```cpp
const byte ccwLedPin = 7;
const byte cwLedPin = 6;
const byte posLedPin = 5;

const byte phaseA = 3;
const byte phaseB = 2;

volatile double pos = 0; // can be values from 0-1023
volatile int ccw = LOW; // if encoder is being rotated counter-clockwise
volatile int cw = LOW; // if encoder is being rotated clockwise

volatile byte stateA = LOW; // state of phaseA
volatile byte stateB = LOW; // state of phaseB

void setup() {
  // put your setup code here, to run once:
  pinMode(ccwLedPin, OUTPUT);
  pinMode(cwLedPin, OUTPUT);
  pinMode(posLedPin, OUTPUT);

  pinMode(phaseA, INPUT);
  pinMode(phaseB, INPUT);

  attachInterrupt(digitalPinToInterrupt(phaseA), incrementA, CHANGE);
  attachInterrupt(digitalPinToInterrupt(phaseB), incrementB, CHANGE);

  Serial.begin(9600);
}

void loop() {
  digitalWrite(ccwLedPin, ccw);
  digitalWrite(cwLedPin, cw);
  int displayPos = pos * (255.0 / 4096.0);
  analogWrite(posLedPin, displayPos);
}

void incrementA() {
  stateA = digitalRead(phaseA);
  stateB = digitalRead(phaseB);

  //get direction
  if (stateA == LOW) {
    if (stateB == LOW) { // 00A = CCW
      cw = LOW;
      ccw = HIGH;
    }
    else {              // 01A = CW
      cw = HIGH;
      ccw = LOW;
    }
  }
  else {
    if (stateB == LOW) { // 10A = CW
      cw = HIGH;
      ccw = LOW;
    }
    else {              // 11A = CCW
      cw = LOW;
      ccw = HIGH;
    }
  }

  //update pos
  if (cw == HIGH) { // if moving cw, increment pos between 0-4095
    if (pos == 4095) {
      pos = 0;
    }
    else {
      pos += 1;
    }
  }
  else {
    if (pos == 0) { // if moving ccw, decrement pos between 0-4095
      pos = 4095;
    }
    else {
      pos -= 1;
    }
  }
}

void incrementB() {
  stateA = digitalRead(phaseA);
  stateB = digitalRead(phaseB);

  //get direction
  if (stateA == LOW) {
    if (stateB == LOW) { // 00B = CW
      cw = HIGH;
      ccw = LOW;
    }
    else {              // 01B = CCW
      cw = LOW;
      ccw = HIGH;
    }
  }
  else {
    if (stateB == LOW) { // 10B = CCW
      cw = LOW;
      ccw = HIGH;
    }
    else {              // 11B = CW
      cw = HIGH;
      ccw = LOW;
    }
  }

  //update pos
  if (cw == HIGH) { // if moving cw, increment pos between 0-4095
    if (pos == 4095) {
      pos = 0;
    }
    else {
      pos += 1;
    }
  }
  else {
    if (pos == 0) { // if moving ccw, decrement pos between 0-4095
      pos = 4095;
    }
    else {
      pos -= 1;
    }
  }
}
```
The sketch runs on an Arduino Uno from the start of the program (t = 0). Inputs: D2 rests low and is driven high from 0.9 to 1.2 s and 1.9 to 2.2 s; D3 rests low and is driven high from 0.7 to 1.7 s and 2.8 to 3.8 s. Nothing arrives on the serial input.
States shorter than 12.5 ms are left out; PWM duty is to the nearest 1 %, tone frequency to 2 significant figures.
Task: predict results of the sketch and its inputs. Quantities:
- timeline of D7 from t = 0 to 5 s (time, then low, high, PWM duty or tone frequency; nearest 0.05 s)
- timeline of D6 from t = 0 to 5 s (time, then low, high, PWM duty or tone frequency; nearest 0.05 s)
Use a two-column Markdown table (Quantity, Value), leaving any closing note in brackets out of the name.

| Quantity | Value |
|---|---|
| timeline of D7 from t = 0 to 5 s | 0 s low; 1.2 s high; 2.2 s low; 3.8 s high |
| timeline of D6 from t = 0 to 5 s | 0 s low; 0.7 s high; 1.2 s low; 2.2 s high; 3.8 s low |
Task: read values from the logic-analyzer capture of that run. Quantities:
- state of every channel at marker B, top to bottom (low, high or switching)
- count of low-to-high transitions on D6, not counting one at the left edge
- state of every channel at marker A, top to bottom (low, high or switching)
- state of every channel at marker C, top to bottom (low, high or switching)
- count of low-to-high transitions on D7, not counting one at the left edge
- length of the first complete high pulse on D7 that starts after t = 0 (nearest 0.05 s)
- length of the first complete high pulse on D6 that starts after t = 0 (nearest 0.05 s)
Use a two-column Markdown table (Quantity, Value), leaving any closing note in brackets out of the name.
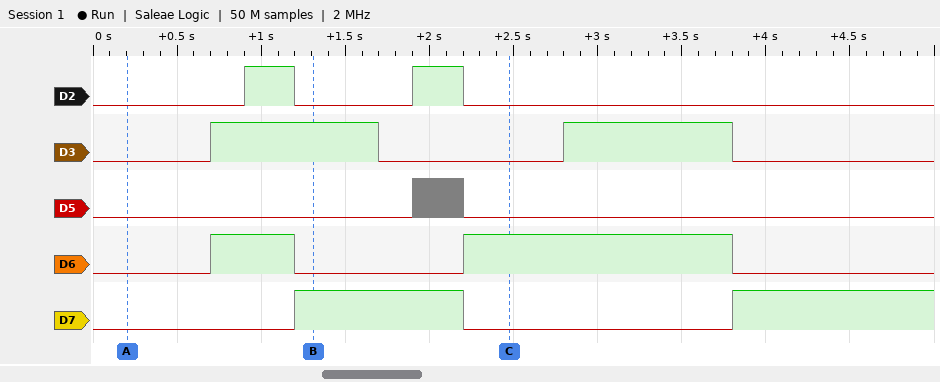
| Quantity | Value |
|---|---|
| state of every channel at marker B, top to bottom | D2 low, D3 high, D5 low, D6 low, D7 high |
| count of low-to-high transitions on D6, not counting one at the left edge | 2 |
| state of every channel at marker A, top to bottom | D2 low, D3 low, D5 low, D6 low, D7 low |
| state of every channel at marker C, top to bottom | D2 low, D3 low, D5 low, D6 high, D7 low |
| count of low-to-high transitions on D7, not counting one at the left edge | 2 |
| length of the first complete high pulse on D7 that starts after t = 0 | 1.00 s |
| length of the first complete high pulse on D6 that starts after t = 0 | 0.50 s |
